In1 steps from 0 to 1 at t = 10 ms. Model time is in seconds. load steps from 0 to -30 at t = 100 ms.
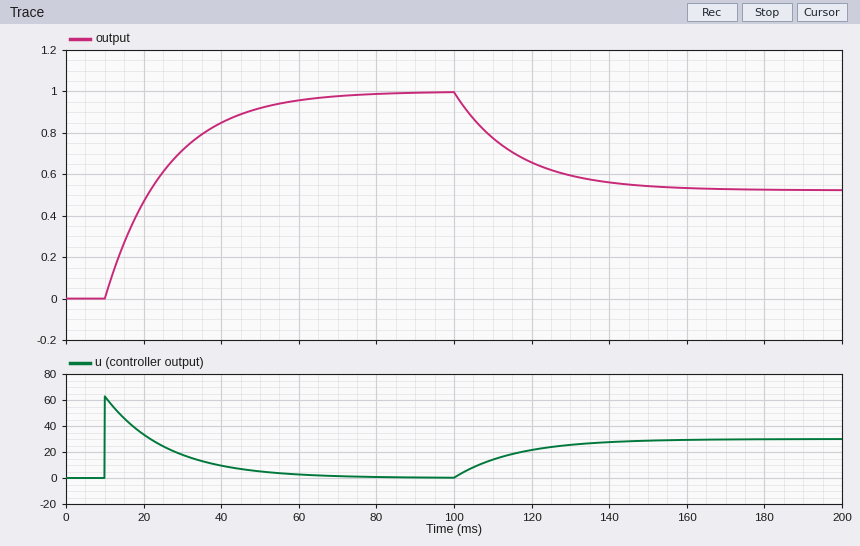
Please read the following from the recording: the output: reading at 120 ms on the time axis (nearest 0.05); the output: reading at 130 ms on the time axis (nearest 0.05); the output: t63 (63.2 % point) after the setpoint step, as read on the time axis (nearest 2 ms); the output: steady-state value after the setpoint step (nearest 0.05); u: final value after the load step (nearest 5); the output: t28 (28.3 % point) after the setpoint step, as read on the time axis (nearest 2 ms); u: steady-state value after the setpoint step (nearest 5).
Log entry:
0.65
0.60
26 ms
1.00
30
16 ms
0
